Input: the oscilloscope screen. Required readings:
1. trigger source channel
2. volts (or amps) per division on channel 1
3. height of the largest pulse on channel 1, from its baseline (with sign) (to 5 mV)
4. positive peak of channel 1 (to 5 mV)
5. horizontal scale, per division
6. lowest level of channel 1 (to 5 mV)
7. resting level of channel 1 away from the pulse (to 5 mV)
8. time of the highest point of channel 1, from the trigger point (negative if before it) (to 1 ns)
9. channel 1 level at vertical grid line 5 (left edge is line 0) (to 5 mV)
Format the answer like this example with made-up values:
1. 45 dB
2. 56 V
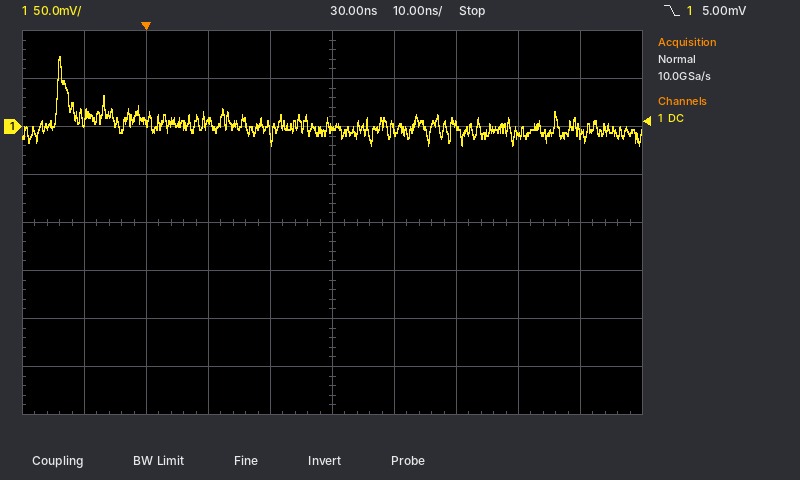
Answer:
1. channel 1
2. 50 mV
3. +75 mV
4. 75 mV
5. 10 ns
6. -20 mV
7. 0 mV
8. -14 ns
9. 0 mV
